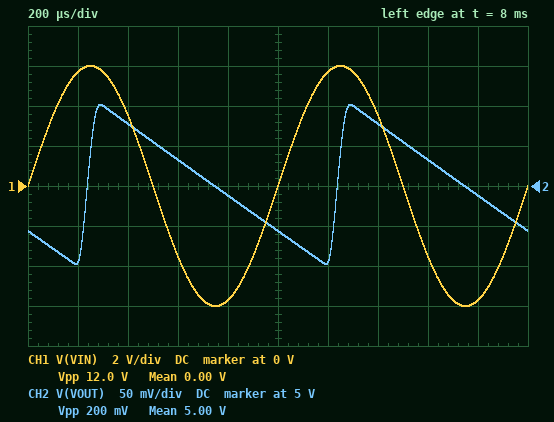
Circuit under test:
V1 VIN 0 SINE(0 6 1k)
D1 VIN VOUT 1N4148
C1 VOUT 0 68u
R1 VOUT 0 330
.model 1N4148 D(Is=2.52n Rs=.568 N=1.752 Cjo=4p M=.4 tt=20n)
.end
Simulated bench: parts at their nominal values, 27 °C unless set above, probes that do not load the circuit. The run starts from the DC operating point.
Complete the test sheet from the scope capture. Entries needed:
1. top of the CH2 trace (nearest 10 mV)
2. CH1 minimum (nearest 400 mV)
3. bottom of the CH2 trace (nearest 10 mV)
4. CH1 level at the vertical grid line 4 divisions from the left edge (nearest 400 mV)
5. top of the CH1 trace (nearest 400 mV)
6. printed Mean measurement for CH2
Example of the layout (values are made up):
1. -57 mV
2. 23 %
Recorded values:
1. 5.10 V
2. -6.0 V
3. 4.90 V
4. -5.6 V
5. 6.0 V
6. 5.00 V
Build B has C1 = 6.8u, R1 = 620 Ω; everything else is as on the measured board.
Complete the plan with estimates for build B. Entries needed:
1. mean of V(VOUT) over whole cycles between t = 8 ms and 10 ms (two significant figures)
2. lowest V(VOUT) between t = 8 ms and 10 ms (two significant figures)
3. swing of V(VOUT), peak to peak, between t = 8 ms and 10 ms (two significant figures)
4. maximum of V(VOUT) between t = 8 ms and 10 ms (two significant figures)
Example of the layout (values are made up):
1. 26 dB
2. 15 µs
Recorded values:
1. 4.8 V
2. 4.3 V
3. 990 mV
4. 5.3 V
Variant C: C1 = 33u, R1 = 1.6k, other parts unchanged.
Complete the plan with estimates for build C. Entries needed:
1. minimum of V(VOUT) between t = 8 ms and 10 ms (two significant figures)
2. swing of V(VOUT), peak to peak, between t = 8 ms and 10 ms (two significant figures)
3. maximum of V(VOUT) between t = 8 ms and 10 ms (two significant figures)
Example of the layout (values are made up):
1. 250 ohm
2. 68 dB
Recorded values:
1. 5.1 V
2. 89 mV
3. 5.2 V
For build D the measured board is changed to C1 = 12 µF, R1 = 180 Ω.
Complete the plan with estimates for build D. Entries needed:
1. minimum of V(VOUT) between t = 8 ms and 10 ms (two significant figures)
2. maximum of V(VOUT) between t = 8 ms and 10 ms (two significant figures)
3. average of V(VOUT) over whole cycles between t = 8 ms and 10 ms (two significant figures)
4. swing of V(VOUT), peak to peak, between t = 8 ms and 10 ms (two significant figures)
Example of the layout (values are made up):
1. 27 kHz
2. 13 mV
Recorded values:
1. 3.5 V
2. 5.2 V
3. 4.4 V
4. 1.7 V
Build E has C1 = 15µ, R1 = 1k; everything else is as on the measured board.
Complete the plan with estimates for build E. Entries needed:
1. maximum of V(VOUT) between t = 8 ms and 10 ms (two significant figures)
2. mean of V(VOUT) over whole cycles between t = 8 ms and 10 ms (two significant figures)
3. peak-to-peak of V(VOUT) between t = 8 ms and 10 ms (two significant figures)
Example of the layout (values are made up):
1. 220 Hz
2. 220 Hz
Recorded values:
1. 5.2 V
2. 5.1 V
3. 310 mV
